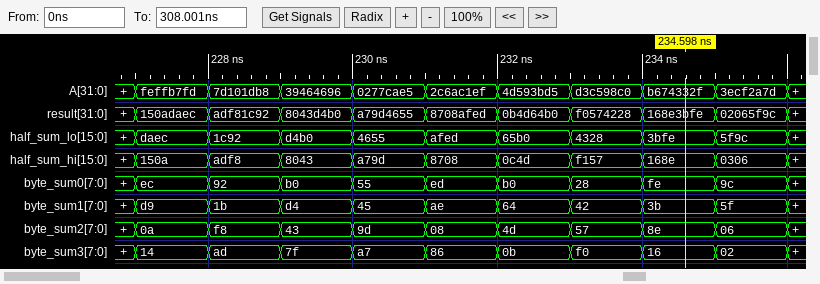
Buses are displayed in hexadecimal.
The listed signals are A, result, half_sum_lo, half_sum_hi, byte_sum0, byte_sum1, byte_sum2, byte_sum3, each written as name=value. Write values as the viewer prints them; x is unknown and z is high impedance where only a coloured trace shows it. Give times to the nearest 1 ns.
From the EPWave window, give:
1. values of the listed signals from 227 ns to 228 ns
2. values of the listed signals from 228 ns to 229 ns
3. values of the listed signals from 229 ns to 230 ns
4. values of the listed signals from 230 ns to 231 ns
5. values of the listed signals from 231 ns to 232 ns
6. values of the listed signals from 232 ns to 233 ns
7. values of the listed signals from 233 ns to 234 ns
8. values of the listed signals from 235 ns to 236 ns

A=feffb7fd, result=150adaec, half_sum_lo=daec, half_sum_hi=150a, byte_sum0=ec, byte_sum1=d9, byte_sum2=0a, byte_sum3=14
A=7d101db8, result=adf81c92, half_sum_lo=1c92, half_sum_hi=adf8, byte_sum0=92, byte_sum1=1b, byte_sum2=f8, byte_sum3=ad
A=39464696, result=8043d4b0, half_sum_lo=d4b0, half_sum_hi=8043, byte_sum0=b0, byte_sum1=d4, byte_sum2=43, byte_sum3=7f
A=0277cae5, result=a79d4655, half_sum_lo=4655, half_sum_hi=a79d, byte_sum0=55, byte_sum1=45, byte_sum2=9d, byte_sum3=a7
A=2c6ac1ef, result=8708afed, half_sum_lo=afed, half_sum_hi=8708, byte_sum0=ed, byte_sum1=ae, byte_sum2=08, byte_sum3=86
A=4d593bd5, result=0b4d64b0, half_sum_lo=65b0, half_sum_hi=0c4d, byte_sum0=b0, byte_sum1=64, byte_sum2=4d, byte_sum3=0b
A=d3c598c0, result=f0574228, half_sum_lo=4328, half_sum_hi=f157, byte_sum0=28, byte_sum1=42, byte_sum2=57, byte_sum3=f0
A=3ecf2a7d, result=02065f9c, half_sum_lo=5f9c, half_sum_hi=0306, byte_sum0=9c, byte_sum1=5f, byte_sum2=06, byte_sum3=02
